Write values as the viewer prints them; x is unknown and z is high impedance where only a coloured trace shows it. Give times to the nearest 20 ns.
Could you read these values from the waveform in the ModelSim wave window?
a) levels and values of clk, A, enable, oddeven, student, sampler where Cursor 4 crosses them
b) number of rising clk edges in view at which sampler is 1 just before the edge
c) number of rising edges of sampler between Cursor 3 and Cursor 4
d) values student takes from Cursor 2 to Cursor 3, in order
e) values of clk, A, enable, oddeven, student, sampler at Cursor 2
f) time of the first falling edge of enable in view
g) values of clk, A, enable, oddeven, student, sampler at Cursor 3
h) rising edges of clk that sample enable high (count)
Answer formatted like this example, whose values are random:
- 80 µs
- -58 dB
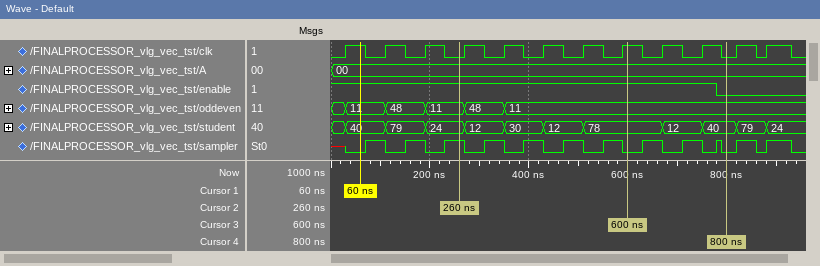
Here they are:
- clk=0, A=00, enable=0, oddeven=11, student=40, sampler=0
- 9
- 3
- 24, 12, 30, 12, 78
- clk=0, A=00, enable=1, oddeven=11, student=24, sampler=1
- 780 ns
- clk=1, A=00, enable=1, oddeven=11, student=78, sampler=0
- 10
